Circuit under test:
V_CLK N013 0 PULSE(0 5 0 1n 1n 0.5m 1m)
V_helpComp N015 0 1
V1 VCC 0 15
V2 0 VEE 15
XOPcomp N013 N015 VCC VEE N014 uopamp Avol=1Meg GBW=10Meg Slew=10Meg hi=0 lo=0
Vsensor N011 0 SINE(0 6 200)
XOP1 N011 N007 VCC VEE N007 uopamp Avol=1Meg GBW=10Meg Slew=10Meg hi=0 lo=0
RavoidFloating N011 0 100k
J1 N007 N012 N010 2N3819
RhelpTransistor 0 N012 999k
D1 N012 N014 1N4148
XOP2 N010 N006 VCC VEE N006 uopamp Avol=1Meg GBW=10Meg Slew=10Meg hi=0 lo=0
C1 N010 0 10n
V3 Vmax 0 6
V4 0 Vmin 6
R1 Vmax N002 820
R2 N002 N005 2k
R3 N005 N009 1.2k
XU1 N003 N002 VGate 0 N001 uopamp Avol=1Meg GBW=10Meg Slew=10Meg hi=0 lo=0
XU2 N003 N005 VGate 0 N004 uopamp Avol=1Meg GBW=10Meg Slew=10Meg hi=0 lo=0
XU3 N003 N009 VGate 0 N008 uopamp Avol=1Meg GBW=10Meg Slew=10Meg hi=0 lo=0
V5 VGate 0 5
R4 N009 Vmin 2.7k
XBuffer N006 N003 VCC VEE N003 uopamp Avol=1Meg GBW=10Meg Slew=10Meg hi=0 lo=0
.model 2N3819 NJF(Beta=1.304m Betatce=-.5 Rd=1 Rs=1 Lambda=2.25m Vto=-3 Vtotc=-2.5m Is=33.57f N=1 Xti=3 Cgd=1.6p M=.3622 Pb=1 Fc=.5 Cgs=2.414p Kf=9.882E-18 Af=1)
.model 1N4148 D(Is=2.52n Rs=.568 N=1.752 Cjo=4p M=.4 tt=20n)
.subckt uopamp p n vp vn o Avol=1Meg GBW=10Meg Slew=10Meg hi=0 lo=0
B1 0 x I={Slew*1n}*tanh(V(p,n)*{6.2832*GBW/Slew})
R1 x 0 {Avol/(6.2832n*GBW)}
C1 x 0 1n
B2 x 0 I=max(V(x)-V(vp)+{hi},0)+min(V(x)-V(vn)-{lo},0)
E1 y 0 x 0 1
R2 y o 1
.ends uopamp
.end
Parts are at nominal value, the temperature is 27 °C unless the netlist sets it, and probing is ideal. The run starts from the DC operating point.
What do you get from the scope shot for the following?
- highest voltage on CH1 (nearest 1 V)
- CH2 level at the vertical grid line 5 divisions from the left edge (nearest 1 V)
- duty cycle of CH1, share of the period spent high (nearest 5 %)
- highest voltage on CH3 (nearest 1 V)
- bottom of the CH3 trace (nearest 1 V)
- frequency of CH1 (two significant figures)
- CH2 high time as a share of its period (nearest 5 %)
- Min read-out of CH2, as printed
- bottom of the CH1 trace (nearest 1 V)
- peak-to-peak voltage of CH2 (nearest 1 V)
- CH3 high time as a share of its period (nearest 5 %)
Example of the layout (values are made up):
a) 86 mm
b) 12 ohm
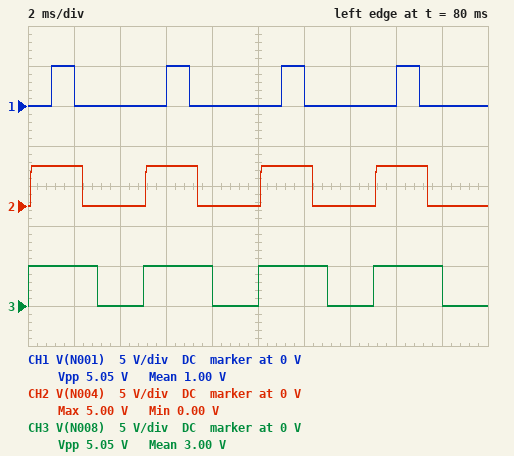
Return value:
a) 5 V
b) 0 V
c) 20 %
d) 5 V
e) 0 V
f) 200 Hz
g) 45 %
h) 0.00 V
i) 0 V
j) 5 V
k) 60 %
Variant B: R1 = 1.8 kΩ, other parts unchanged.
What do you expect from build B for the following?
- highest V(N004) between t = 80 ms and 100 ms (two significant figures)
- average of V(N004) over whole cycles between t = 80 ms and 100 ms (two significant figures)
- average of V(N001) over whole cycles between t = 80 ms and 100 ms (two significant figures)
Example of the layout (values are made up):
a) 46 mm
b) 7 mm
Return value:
a) 5.0 V
b) 2.5 V
c) 1.1 V
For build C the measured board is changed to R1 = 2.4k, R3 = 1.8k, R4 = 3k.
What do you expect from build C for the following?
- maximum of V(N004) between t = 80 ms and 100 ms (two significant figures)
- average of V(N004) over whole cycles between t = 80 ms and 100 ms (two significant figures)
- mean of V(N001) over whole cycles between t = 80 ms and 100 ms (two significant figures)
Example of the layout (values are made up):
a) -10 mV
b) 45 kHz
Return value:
a) 5.0 V
b) 2.4 V
c) 1.7 V
